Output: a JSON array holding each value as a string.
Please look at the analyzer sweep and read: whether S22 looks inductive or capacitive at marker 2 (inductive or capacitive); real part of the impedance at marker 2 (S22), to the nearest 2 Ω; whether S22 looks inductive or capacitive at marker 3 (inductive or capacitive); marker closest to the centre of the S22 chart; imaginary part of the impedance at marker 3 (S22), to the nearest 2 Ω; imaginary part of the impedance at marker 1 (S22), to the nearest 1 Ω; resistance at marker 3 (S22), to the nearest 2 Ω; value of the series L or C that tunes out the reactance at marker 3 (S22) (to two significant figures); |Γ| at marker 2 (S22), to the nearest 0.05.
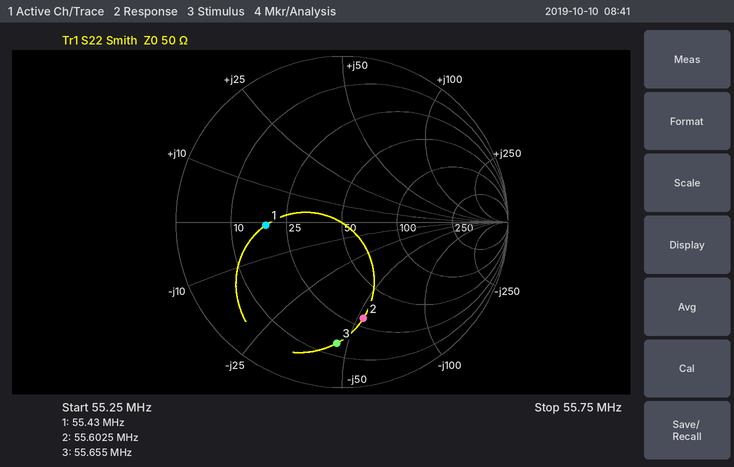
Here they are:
["capacitive", "30 Ω", "capacitive", "marker 1", "-46 Ω", "-1 Ω", "14 Ω", "130 nH", "0.60"]
